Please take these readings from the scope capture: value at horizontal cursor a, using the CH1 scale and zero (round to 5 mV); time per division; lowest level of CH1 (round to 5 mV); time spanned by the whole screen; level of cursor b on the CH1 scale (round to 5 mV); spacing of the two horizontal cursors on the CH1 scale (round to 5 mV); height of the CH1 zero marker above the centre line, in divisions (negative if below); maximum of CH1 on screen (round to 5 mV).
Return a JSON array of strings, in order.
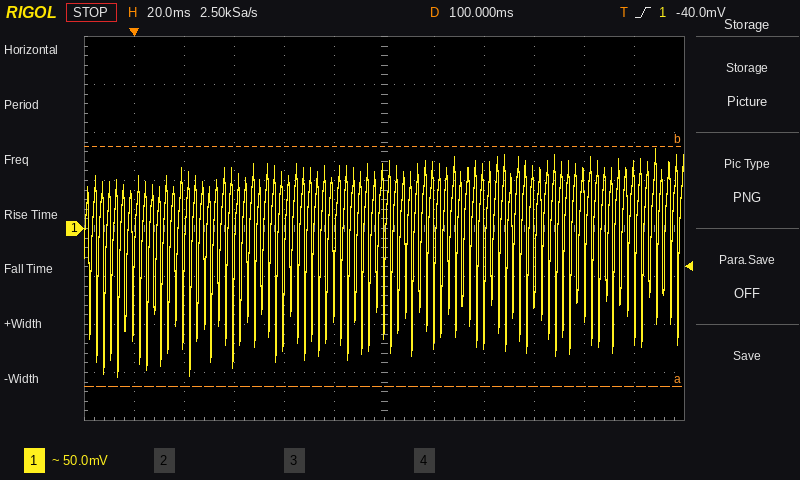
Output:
["-165 mV", "20 ms", "-155 mV", "240 ms", "85 mV", "250 mV", "0.0 div", "85 mV"]
